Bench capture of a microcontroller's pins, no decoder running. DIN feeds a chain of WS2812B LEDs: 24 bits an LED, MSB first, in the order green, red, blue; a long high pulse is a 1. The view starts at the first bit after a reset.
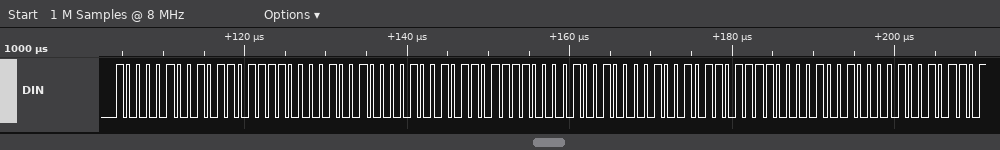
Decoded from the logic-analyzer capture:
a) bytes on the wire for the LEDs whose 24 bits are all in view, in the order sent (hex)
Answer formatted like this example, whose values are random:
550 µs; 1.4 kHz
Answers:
84 B7 84 84 B7 84 84 B7 84
